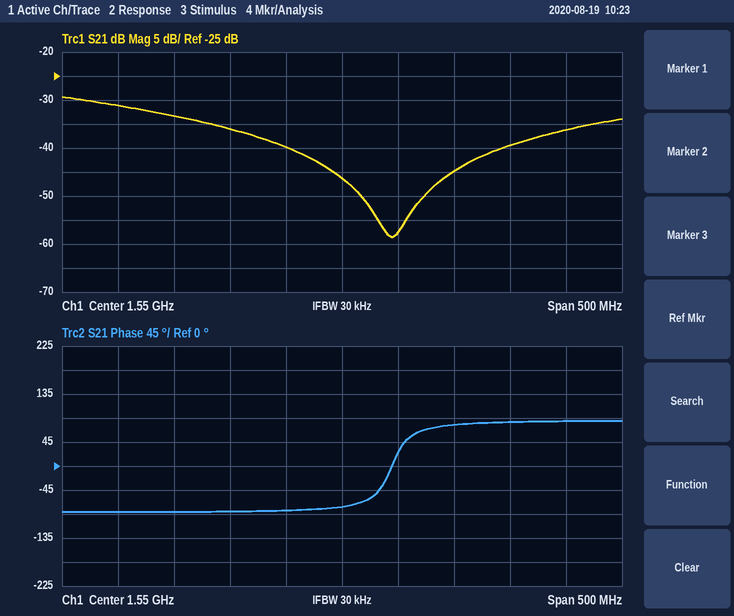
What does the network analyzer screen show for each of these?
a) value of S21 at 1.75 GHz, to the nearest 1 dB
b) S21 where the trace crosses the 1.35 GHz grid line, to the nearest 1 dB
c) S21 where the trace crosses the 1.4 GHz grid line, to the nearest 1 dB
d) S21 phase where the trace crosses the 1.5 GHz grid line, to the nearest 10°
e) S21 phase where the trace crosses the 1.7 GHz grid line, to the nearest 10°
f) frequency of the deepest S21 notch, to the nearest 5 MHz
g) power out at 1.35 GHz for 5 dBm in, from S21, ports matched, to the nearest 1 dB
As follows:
-36 dB
-31 dB
-33 dB
-80°
80°
1.595 GHz
-26 dBm
